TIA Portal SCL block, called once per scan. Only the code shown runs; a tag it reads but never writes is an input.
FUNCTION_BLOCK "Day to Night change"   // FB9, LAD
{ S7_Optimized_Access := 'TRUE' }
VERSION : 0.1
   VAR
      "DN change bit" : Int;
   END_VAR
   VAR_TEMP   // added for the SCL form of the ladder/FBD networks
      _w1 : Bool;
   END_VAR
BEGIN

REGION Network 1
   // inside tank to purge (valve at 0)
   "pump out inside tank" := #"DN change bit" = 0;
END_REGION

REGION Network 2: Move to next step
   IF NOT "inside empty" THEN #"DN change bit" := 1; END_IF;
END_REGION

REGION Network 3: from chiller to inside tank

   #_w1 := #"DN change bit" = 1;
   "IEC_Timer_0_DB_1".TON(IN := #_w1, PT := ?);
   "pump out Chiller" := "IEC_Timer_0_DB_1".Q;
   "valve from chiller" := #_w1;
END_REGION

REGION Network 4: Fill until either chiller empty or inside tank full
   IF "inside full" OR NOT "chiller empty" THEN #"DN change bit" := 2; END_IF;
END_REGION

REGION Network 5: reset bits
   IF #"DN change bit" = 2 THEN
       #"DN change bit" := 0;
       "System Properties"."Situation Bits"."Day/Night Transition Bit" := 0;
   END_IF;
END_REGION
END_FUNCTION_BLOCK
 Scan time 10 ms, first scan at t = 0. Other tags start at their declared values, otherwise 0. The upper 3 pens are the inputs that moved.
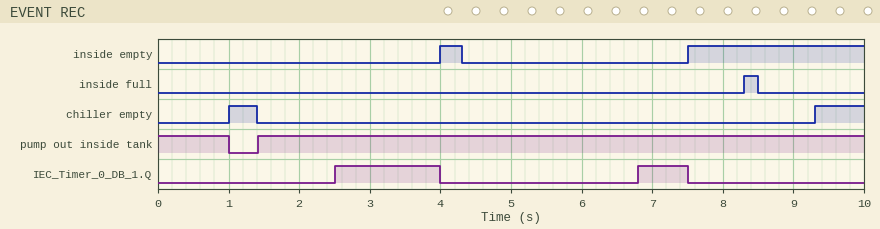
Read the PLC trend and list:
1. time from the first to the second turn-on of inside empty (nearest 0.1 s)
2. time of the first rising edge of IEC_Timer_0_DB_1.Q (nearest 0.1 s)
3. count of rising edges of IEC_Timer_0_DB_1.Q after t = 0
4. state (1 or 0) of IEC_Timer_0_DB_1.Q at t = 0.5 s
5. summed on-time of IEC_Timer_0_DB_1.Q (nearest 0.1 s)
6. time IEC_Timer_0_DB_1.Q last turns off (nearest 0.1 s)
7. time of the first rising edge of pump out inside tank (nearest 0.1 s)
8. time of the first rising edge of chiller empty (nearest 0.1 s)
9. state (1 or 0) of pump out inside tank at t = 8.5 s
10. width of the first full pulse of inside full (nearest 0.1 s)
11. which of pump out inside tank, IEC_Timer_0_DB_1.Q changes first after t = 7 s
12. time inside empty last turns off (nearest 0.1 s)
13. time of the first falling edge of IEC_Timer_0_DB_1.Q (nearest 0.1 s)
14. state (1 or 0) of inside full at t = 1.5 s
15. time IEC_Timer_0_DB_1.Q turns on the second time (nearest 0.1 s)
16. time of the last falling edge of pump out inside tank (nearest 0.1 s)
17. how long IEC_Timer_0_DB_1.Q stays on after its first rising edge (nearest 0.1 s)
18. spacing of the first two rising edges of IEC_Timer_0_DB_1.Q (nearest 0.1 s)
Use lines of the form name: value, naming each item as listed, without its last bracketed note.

time from the first to the second turn-on of inside empty: 3.5 s
time of the first rising edge of IEC_Timer_0_DB_1.Q: 2.5 s
count of rising edges of IEC_Timer_0_DB_1.Q after t = 0: 2
state (1 or 0) of IEC_Timer_0_DB_1.Q at t = 0.5 s: 0
summed on-time of IEC_Timer_0_DB_1.Q: 2.2 s
time IEC_Timer_0_DB_1.Q last turns off: 7.5 s
time of the first rising edge of pump out inside tank: 1.4 s
time of the first rising edge of chiller empty: 1.0 s
state (1 or 0) of pump out inside tank at t = 8.5 s: 1
width of the first full pulse of inside full: 0.2 s
which of pump out inside tank, IEC_Timer_0_DB_1.Q changes first after t = 7 s: IEC_Timer_0_DB_1.Q
time inside empty last turns off: 4.3 s
time of the first falling edge of IEC_Timer_0_DB_1.Q: 4.0 s
state (1 or 0) of inside full at t = 1.5 s: 0
time IEC_Timer_0_DB_1.Q turns on the second time: 6.8 s
time of the last falling edge of pump out inside tank: 1.0 s
how long IEC_Timer_0_DB_1.Q stays on after its first rising edge: 1.5 s
spacing of the first two rising edges of IEC_Timer_0_DB_1.Q: 4.3 s
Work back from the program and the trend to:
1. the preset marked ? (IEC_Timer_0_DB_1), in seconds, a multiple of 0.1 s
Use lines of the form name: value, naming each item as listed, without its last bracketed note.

the preset marked ? (IEC_Timer_0_DB_1), in seconds, a multiple of 0.1 s: 2.5 s
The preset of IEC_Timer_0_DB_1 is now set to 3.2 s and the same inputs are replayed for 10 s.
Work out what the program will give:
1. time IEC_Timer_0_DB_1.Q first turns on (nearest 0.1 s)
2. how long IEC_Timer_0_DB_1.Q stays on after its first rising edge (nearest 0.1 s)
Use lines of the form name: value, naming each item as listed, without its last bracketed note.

time IEC_Timer_0_DB_1.Q first turns on: 3.2 s
how long IEC_Timer_0_DB_1.Q stays on after its first rising edge: 0.8 s
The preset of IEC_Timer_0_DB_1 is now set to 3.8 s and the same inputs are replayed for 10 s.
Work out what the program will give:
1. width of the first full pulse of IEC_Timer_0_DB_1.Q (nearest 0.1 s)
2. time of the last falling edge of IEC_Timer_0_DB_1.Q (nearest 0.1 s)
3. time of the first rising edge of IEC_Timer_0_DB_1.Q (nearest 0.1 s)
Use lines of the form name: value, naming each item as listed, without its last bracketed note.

width of the first full pulse of IEC_Timer_0_DB_1.Q: 0.2 s
time of the last falling edge of IEC_Timer_0_DB_1.Q: 4.0 s
time of the first rising edge of IEC_Timer_0_DB_1.Q: 3.8 s
